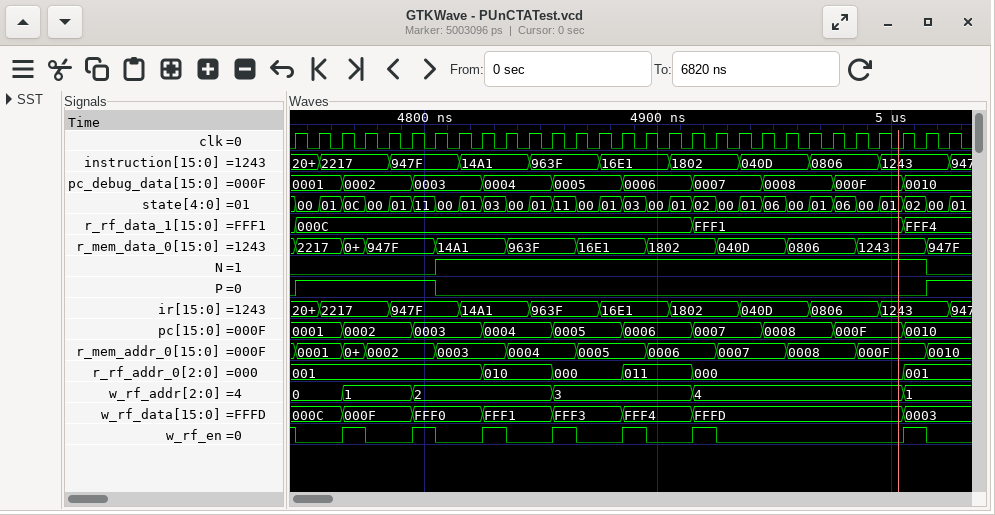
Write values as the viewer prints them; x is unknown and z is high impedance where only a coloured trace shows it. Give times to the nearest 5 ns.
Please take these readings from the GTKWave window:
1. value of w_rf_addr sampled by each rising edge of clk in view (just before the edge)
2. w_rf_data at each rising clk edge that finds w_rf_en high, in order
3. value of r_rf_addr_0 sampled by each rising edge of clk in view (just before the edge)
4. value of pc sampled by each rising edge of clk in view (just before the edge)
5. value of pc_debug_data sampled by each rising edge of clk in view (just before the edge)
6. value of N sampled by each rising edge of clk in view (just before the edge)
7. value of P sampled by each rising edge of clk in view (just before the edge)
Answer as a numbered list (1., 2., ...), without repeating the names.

1. 0, 0, 0, 1, 1, 1, 2, 2, 2, 2, 2, 2, 3, 3, 3, 3, 3, 3, 4, 4, 4, 4, 4, 4, 4, 4, 4, 1, 1
2. 000C, 000F, FFF0, FFF1, FFF3, FFF4, FFFD, 0003
3. 001, 001, 001, 001, 001, 001, 001, 001, 001, 010, 010, 010, 000, 000, 000, 011, 011, 011, 000, 000, 000, 000, 000, 000, 000, 000, 000, 001, 001
4. 0001, 0001, 0001, 0002, 0002, 0002, 0003, 0003, 0003, 0004, 0004, 0004, 0005, 0005, 0005, 0006, 0006, 0006, 0007, 0007, 0007, 0008, 0008, 0008, 000F, 000F, 000F, 0010, 0010
5. 0001, 0001, 0001, 0002, 0002, 0002, 0003, 0003, 0003, 0004, 0004, 0004, 0005, 0005, 0005, 0006, 0006, 0006, 0007, 0007, 0007, 0008, 0008, 0008, 000F, 000F, 000F, 0010, 0010
6. 0 0 0 0 0 0 0 1 1 1 1 1 1 1 1 1 1 1 1 1 1 1 1 1 1 1 1 1 0
7. 0 1 1 1 1 1 1 0 0 0 0 0 0 0 0 0 0 0 0 0 0 0 0 0 0 0 0 0 1
